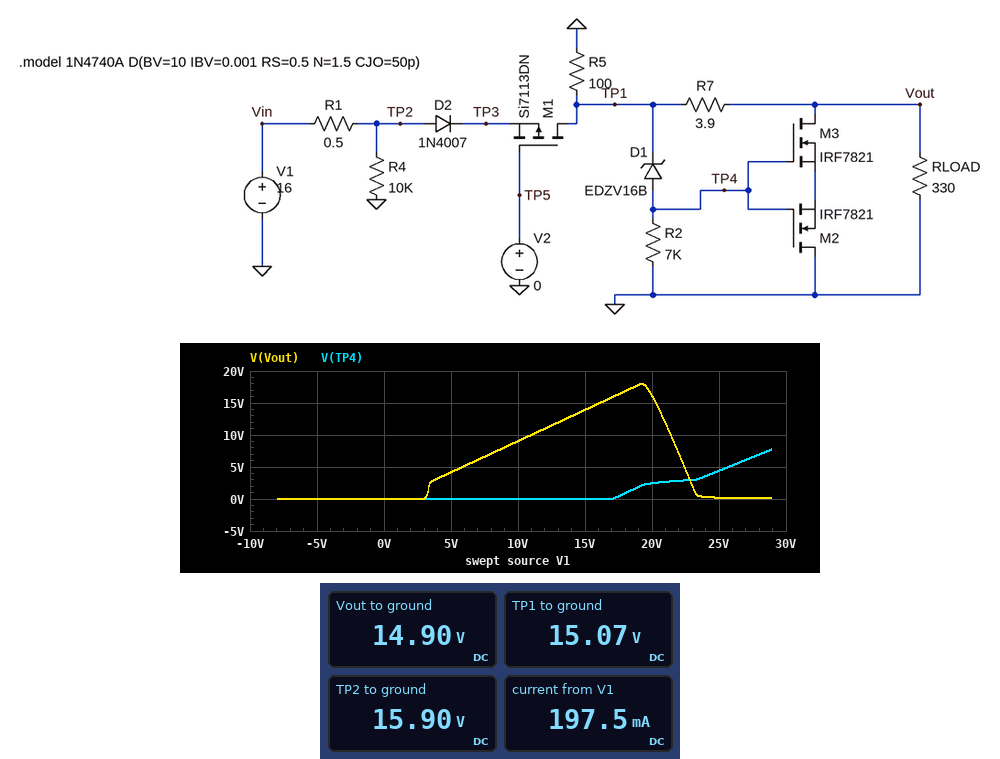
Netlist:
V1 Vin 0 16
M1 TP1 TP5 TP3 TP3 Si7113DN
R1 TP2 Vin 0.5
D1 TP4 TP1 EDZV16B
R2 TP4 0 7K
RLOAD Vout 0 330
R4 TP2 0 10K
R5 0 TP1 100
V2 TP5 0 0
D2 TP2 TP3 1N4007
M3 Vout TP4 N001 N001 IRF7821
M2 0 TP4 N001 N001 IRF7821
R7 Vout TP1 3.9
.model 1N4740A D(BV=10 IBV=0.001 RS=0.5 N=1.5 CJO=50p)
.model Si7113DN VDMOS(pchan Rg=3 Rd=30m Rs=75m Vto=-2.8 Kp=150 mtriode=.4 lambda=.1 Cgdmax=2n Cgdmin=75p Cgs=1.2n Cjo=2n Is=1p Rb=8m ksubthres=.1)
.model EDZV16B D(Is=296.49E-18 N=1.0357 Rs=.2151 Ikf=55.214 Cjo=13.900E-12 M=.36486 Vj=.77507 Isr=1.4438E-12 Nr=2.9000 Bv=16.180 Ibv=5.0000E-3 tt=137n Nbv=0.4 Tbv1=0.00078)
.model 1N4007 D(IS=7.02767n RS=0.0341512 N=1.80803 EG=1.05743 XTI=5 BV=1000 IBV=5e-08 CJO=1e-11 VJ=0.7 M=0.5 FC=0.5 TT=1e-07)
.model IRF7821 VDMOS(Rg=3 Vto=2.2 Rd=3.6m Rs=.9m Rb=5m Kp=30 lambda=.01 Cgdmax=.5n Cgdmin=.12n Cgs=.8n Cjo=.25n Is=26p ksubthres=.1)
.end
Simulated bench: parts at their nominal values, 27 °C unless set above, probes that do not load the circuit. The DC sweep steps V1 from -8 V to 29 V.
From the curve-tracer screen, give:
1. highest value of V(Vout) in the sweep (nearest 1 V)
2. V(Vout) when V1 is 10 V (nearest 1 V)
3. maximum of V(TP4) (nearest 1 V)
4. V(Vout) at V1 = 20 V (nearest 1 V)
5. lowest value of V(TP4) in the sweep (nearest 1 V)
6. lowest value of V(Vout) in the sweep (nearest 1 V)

18 V
9 V
8 V
16 V
0 V
0 V
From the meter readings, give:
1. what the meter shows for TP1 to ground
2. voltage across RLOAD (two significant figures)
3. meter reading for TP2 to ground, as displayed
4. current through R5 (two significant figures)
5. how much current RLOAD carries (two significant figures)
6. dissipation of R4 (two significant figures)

15.07 V
15 V
15.90 V
150 mA
45 mA
25 mW
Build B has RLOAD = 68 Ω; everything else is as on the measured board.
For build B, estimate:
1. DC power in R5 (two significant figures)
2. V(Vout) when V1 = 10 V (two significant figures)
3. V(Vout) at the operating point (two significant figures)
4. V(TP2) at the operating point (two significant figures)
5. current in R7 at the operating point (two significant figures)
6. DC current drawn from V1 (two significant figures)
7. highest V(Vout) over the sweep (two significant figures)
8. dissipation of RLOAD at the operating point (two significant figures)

2.2 W
8.6 V
14 V
16 V
210 mA
360 mA
17 V
2.9 W
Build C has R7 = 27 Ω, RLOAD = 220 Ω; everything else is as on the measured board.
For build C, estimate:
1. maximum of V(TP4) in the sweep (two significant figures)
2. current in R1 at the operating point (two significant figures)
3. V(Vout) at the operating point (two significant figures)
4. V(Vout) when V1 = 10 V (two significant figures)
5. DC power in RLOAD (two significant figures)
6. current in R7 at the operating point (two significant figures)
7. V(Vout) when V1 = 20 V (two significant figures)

11 V
210 mA
13 V
8.1 V
820 mW
61 mA
2.2 V
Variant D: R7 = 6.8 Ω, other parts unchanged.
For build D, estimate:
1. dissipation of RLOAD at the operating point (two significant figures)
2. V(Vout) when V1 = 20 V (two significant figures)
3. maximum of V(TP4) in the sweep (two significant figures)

660 mW
14 V
9.3 V
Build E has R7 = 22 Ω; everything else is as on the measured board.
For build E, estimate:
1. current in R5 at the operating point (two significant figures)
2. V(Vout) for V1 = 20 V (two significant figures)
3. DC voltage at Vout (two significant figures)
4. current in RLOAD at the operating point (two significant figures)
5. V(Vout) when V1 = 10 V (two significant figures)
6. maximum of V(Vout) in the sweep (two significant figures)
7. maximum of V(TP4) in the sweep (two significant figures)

150 mA
5.2 V
14 V
43 mA
8.6 V
17 V
11 V
